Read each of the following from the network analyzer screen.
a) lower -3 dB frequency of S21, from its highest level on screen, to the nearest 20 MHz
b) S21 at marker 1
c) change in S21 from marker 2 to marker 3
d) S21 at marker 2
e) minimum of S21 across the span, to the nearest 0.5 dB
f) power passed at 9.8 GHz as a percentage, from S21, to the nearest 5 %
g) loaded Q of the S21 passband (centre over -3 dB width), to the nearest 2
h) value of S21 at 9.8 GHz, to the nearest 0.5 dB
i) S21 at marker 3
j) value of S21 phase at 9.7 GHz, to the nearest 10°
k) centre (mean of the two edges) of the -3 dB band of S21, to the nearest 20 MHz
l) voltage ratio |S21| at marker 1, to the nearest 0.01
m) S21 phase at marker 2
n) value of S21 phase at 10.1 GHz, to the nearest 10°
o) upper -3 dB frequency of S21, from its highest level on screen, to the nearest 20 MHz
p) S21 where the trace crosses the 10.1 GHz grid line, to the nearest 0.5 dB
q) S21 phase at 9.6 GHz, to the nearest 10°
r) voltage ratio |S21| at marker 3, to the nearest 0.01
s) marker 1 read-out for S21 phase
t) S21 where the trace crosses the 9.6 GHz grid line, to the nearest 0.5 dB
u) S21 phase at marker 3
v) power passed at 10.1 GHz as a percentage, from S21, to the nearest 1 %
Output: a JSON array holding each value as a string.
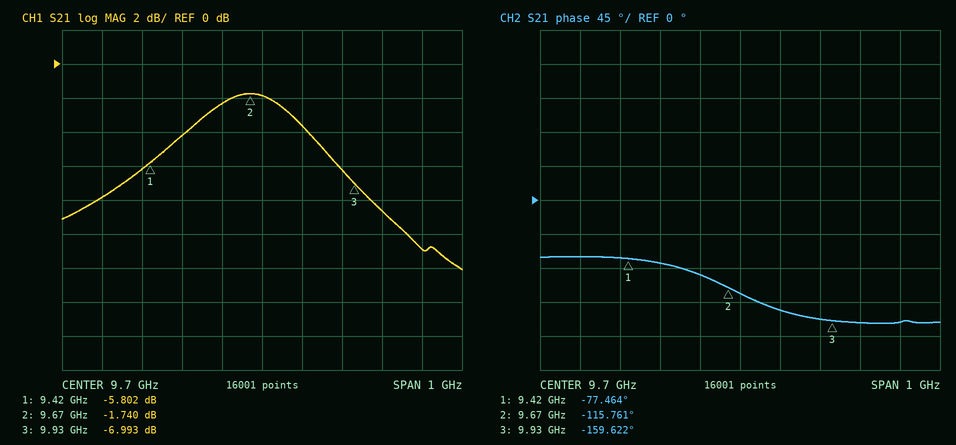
["9.48 GHz", "-5.802 dB", "-5.253 dB", "-1.740 dB", "-12.0 dB", "45 %", "26", "-3.5 dB", "-6.993 dB", "-120°", "9.66 GHz", "0.51", "-115.761°", "-160°", "9.84 GHz", "-11.0 dB", "-100°", "0.45", "-77.464°", "-2.5 dB", "-159.622°", "8 %"]
